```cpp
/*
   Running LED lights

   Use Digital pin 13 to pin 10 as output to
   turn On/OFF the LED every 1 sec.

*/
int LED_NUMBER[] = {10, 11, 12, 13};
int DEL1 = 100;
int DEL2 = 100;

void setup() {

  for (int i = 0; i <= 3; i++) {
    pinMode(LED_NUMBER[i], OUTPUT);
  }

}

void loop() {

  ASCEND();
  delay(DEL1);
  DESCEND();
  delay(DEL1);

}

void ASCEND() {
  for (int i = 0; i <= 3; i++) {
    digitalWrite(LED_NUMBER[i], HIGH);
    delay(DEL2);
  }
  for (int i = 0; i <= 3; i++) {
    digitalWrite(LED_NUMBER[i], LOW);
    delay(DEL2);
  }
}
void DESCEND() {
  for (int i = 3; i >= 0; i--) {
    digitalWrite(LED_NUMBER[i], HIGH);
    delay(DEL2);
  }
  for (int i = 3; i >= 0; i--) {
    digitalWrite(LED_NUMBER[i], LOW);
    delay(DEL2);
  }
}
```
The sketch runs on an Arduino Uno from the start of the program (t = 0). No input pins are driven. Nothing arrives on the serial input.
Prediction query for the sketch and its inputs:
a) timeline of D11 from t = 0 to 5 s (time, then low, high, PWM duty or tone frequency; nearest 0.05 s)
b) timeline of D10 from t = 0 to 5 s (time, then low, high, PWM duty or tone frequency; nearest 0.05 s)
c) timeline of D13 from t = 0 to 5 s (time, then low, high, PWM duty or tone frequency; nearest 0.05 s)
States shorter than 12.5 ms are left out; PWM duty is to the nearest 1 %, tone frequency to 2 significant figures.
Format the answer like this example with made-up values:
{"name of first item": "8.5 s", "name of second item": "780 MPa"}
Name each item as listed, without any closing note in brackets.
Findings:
{"timeline of D11 from t = 0 to 5 s": "0 s low; 0.1 s high; 0.5 s low; 1.1 s high; 1.5 s low; 1.9 s high; 2.3 s low; 2.9 s high; 3.3 s low; 3.7 s high; 4.1 s low; 4.7 s high", "timeline of D10 from t = 0 to 5 s": "0 s high; 0.4 s low; 1.2 s high; 1.6 s low; 1.8 s high; 2.2 s low; 3 s high; 3.4 s low; 3.6 s high; 4 s low; 4.8 s high", "timeline of D13 from t = 0 to 5 s": "0 s low; 0.3 s high; 0.7 s low; 0.9 s high; 1.3 s low; 2.1 s high; 2.5 s low; 2.7 s high; 3.1 s low; 3.9 s high; 4.3 s low; 4.5 s high; 4.9 s low"}
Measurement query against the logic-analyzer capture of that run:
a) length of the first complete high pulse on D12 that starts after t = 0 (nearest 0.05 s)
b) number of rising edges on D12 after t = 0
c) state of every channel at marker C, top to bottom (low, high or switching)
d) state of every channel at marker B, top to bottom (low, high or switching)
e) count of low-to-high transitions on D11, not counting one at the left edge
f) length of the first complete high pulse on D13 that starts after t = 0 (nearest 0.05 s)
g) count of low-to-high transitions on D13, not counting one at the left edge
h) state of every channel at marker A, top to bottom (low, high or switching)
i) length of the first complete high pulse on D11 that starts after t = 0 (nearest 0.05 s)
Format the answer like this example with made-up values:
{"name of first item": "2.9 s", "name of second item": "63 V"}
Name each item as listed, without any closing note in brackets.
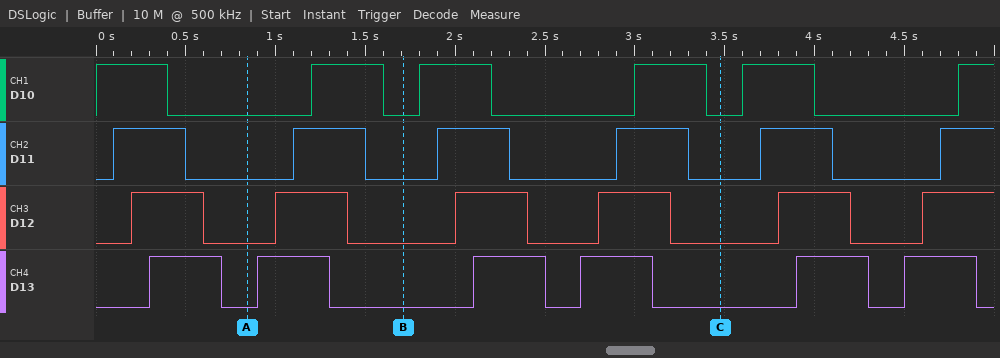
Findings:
{"length of the first complete high pulse on D12 that starts after t = 0": "0.40 s", "number of rising edges on D12 after t = 0": "6", "state of every channel at marker C, top to bottom": "D10 low, D11 low, D12 low, D13 low", "state of every channel at marker B, top to bottom": "D10 low, D11 low, D12 low, D13 low", "count of low-to-high transitions on D11, not counting one at the left edge": "6", "length of the first complete high pulse on D13 that starts after t = 0": "0.40 s", "count of low-to-high transitions on D13, not counting one at the left edge": "6", "state of every channel at marker A, top to bottom": "D10 low, D11 low, D12 low, D13 low", "length of the first complete high pulse on D11 that starts after t = 0": "0.40 s"}
